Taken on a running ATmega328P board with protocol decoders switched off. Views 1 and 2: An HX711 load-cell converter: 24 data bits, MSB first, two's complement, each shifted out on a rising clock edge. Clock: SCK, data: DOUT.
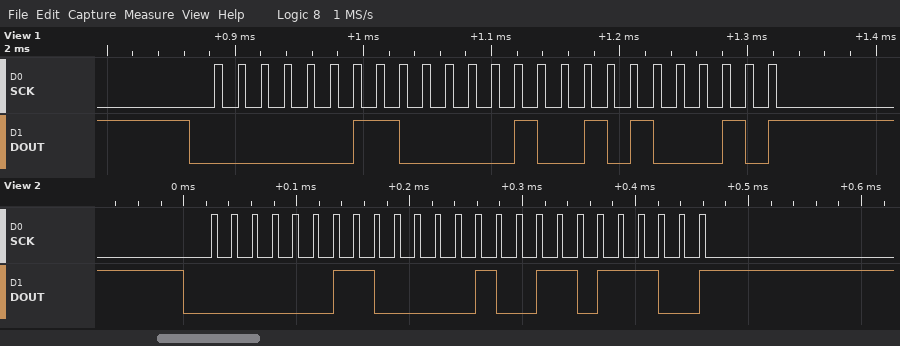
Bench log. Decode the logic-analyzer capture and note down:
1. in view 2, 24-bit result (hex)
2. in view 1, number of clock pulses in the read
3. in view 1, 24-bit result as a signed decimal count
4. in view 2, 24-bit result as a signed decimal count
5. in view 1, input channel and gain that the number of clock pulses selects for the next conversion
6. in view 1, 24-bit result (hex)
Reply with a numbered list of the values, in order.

1. 0x0304DC
2. 25
3. 197794
4. 197852
5. channel A, gain 128
6. 0x0304A2
